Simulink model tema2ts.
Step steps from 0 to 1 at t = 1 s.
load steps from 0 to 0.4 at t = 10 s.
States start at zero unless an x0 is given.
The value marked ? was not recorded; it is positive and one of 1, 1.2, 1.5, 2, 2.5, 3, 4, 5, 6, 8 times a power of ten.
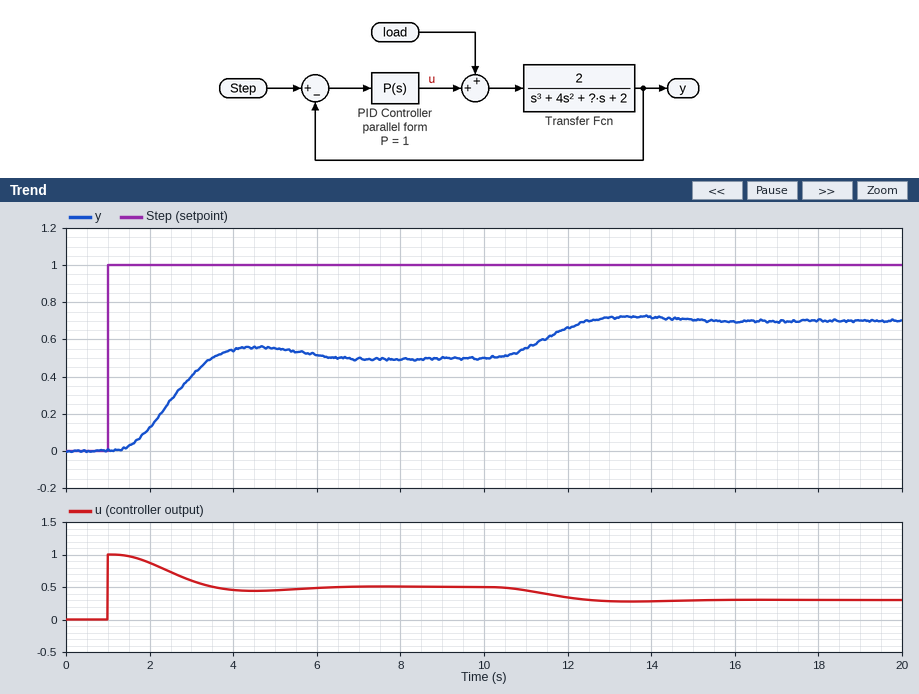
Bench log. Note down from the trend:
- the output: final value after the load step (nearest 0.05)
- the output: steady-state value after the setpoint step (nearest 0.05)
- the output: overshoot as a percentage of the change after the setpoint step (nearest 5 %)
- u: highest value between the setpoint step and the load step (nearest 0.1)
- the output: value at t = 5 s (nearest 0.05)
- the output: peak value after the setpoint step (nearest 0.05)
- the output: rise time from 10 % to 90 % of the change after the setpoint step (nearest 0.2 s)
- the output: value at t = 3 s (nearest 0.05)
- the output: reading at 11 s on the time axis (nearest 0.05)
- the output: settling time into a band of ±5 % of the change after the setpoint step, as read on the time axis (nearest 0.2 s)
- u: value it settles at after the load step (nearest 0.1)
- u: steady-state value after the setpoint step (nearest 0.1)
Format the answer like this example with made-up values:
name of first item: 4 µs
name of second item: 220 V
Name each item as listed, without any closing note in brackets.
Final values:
the output: final value after the load step: 0.70
the output: steady-state value after the setpoint step: 0.50
the output: overshoot as a percentage of the change after the setpoint step: 10 %
u: highest value between the setpoint step and the load step: 1.0
the output: value at t = 5 s: 0.55
the output: peak value after the setpoint step: 0.55
the output: rise time from 10 % to 90 % of the change after the setpoint step: 1.6 s
the output: value at t = 3 s: 0.40
the output: reading at 11 s on the time axis: 0.55
the output: settling time into a band of ±5 % of the change after the setpoint step, as read on the time axis: 5.8 s
u: value it settles at after the load step: 0.3
u: steady-state value after the setpoint step: 0.5
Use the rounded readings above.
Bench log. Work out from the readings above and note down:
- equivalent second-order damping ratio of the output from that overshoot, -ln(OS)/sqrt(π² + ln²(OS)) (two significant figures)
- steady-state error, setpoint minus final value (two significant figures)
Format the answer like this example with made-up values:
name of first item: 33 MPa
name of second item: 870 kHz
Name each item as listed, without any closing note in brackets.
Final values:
equivalent second-order damping ratio of the output from that overshoot, -ln(OS)/sqrt(π² + ln²(OS)): 0.59
steady-state error, setpoint minus final value: 0.50
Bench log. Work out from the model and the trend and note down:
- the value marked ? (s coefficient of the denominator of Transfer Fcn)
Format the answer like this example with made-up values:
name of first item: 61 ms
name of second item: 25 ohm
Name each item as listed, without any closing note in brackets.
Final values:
the value marked ?: 5
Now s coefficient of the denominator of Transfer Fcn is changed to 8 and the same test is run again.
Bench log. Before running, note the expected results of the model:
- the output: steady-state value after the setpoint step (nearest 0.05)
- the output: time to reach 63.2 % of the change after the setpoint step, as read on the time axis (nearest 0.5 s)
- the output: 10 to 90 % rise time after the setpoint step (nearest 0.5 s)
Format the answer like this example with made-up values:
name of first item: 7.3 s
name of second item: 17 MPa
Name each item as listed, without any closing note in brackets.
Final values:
the output: steady-state value after the setpoint step: 0.50
the output: time to reach 63.2 % of the change after the setpoint step, as read on the time axis: 3.0 s
the output: 10 to 90 % rise time after the setpoint step: 3.0 s
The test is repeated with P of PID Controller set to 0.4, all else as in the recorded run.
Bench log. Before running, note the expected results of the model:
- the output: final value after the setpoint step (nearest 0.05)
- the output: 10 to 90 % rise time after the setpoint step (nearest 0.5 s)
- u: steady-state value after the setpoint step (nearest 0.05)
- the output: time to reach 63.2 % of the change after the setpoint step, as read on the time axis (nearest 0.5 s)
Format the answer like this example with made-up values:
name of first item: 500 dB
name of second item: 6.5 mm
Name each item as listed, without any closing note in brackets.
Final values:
the output: final value after the setpoint step: 0.30
the output: 10 to 90 % rise time after the setpoint step: 2.5 s
u: steady-state value after the setpoint step: 0.30
the output: time to reach 63.2 % of the change after the setpoint step, as read on the time axis: 3.0 s
